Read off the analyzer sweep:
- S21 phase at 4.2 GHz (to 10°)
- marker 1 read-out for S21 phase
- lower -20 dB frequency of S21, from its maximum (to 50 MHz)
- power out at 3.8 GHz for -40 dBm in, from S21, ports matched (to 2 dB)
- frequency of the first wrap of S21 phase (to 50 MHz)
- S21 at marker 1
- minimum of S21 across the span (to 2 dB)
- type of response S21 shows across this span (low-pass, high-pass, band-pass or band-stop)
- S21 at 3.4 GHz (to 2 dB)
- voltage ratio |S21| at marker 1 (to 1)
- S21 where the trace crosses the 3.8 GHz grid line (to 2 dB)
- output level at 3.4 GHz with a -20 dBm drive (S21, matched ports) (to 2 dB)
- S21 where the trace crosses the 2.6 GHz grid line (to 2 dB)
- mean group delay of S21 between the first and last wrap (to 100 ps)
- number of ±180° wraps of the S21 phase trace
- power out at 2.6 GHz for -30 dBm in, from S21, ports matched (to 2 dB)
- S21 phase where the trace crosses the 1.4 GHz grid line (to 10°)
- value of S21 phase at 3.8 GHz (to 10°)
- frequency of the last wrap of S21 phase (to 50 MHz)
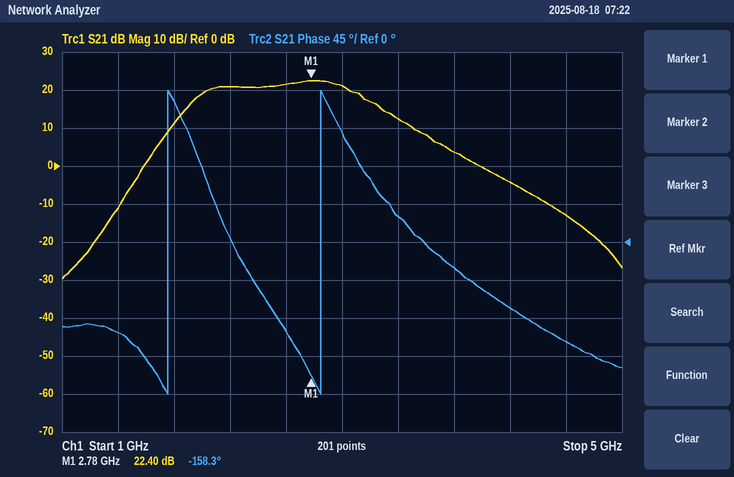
-80°
-158.3°
1.65 GHz
-36 dBm
1.75 GHz
22.40 dB
-30 dB
band-pass
12 dB
13
4 dB
-8 dBm
22 dB
900 ps
2
-8 dBm
-110°
-30°
2.85 GHz
